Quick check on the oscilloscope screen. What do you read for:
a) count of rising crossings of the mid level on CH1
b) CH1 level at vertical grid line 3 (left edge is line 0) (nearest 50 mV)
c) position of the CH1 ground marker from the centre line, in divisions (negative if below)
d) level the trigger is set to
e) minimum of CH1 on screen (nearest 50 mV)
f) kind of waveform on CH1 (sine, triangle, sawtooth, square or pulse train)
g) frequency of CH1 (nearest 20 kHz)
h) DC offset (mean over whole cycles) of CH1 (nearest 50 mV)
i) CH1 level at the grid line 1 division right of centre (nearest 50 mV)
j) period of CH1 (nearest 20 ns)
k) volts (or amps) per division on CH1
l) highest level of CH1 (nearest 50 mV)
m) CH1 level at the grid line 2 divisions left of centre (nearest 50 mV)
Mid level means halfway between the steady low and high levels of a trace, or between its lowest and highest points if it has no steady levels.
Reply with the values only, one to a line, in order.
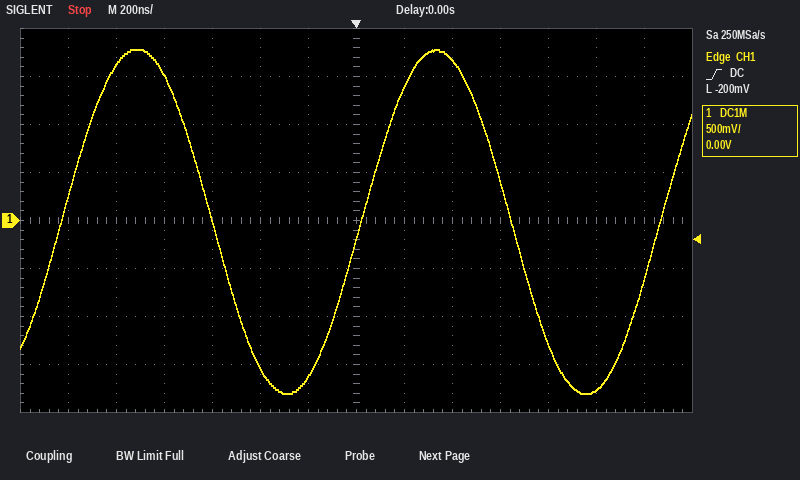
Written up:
3
1.50 V
0.0 div
-200 mV
-1.80 V
sine
800 kHz
0 mV
1.40 V
1.24 µs
500 mV
1.80 V
-1.55 V
